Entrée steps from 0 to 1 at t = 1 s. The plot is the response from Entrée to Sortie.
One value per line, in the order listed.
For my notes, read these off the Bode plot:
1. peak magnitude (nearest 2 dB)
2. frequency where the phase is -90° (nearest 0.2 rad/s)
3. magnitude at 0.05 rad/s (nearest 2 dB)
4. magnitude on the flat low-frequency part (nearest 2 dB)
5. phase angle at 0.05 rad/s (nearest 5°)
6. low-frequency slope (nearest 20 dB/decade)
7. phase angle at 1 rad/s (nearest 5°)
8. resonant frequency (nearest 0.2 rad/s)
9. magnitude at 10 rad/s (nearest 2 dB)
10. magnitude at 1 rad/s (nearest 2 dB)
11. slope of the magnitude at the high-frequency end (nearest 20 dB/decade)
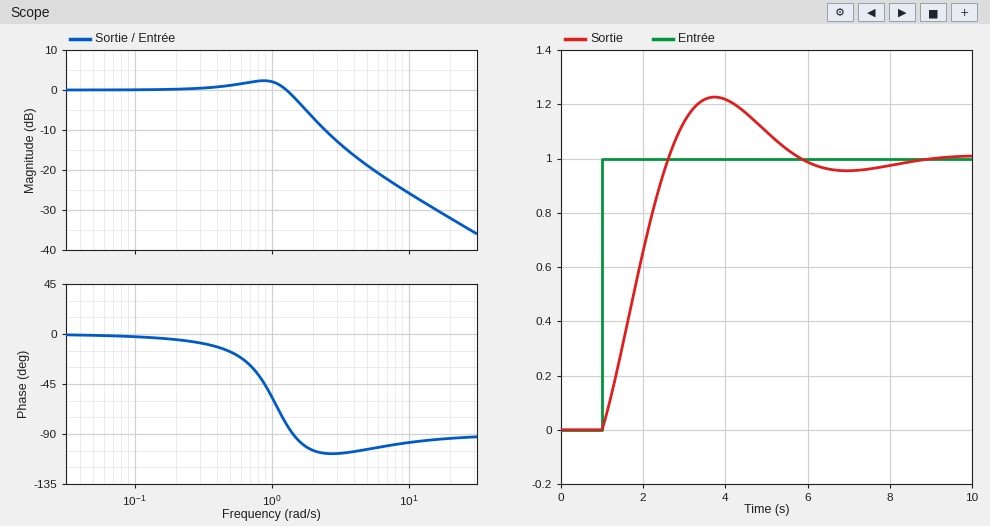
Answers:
2 dB
1.4 rad/s
0 dB
0 dB
0°
0 dB/decade
-55°
0.8 rad/s
-26 dB
2 dB
-20 dB/decade
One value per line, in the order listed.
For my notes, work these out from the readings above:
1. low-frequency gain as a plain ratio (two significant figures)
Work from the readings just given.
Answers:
1.0
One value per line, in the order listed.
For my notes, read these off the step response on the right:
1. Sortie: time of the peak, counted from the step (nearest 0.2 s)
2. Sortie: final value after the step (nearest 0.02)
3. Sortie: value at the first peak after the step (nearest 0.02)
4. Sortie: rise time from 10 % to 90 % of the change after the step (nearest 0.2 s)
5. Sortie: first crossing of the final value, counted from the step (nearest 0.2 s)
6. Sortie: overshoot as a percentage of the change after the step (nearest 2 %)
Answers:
2.8 s
1.00
1.22
1.2 s
1.6 s
22 %
